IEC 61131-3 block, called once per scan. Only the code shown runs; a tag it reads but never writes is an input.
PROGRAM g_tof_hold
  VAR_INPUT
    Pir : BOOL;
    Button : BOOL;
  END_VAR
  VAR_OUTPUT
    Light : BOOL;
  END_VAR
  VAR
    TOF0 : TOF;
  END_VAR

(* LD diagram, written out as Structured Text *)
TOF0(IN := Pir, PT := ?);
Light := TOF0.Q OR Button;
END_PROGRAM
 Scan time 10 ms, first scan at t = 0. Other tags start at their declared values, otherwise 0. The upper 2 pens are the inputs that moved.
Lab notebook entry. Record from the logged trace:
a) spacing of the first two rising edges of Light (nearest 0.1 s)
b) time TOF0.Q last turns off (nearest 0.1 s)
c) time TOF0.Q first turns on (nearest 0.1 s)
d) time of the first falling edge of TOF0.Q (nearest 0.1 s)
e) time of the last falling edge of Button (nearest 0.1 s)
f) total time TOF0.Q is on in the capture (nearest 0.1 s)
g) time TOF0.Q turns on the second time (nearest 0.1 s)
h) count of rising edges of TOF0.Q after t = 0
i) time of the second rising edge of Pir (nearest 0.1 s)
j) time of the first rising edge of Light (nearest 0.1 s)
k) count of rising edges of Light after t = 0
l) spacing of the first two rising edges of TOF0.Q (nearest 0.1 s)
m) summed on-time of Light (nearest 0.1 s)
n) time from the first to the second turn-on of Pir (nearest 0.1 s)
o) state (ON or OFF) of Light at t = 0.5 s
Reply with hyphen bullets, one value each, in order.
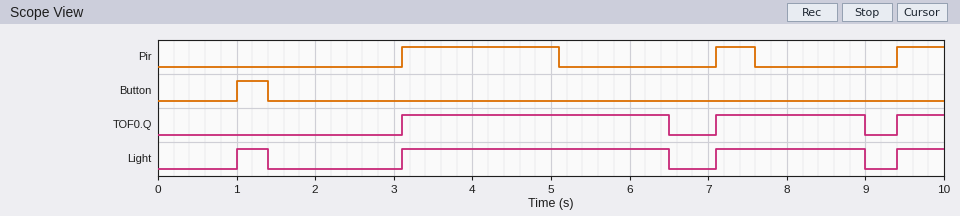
- 2.1 s
- 9.0 s
- 3.1 s
- 6.5 s
- 1.4 s
- 5.9 s
- 7.1 s
- 3
- 7.1 s
- 1.0 s
- 4
- 4.0 s
- 6.3 s
- 4.0 s
- OFF
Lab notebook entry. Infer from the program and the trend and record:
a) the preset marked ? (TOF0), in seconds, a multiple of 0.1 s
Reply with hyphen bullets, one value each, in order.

- 1.4 s
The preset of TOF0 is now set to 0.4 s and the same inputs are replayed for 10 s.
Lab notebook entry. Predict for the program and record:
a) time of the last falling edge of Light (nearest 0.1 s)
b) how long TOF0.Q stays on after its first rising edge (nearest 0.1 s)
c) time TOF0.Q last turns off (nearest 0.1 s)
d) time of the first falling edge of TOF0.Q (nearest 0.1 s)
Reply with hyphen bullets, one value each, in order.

- 8.0 s
- 2.4 s
- 8.0 s
- 5.5 s
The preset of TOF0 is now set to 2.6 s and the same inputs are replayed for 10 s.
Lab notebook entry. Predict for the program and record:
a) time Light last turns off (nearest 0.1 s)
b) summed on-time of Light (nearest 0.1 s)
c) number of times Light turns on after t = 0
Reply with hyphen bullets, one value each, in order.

- 1.4 s
- 7.3 s
- 2
